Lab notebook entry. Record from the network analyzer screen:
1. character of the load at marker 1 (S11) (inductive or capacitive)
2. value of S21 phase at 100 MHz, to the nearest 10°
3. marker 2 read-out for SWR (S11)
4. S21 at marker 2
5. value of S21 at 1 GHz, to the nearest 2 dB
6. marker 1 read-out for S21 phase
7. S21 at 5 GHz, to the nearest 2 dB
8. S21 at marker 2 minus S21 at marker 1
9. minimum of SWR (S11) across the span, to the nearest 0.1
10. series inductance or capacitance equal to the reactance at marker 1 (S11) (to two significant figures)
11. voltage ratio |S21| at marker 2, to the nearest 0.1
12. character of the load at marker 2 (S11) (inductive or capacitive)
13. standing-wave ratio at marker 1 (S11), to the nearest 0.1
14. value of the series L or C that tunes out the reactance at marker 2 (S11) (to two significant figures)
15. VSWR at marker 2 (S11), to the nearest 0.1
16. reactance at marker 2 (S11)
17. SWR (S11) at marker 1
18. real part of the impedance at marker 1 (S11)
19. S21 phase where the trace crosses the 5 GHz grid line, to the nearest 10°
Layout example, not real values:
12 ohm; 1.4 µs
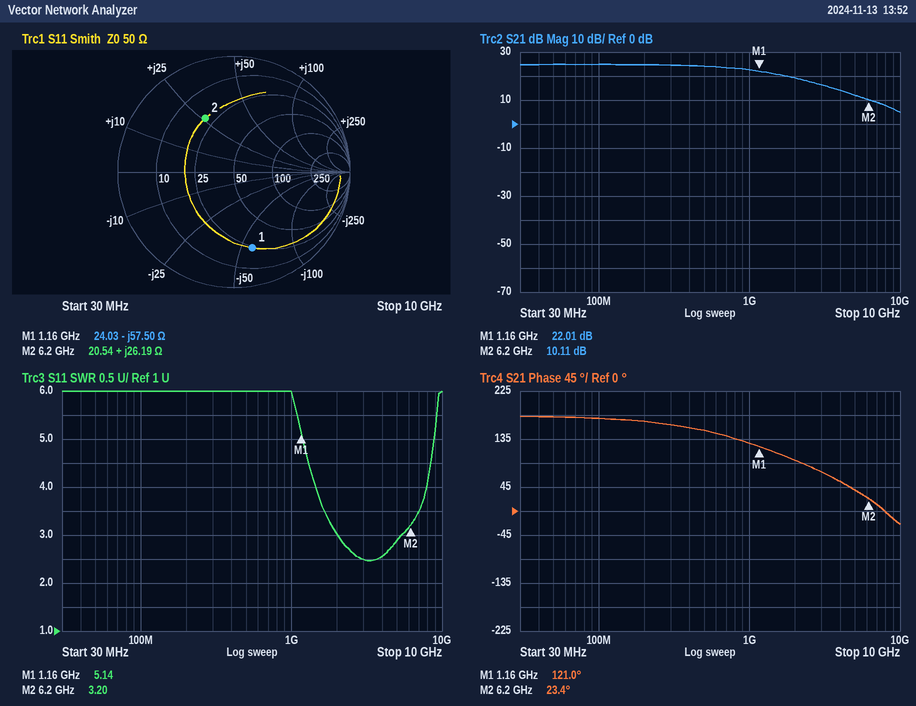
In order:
capacitive; 170°; 3.20; 10.11 dB; 22 dB; 121.0°; 12 dB; -11.90 dB; 2.5; 2.4 pF; 3.2; inductive; 5.1; 980 fF; 3.2; +26.19 Ω; 5.14; 24.03 Ω; 40°
